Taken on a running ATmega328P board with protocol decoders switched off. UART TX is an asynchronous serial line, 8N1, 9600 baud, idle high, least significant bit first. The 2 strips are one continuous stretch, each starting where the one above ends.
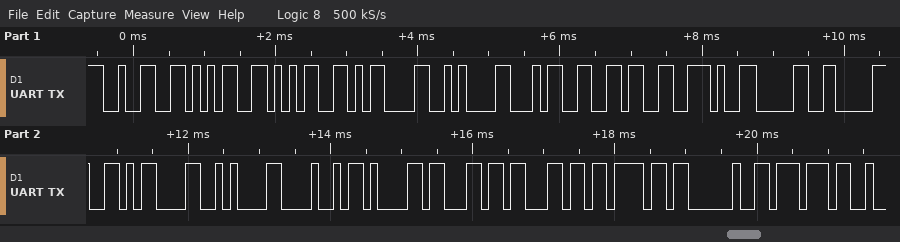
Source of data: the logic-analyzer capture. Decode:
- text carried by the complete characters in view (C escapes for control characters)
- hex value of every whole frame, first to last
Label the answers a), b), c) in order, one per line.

a) "255\r\n46.00\r\nHallo w"
b) 32 35 35 0D 0A 34 36 2E 30 30 0D 0A 48 61 6C 6C 6F 20 77
